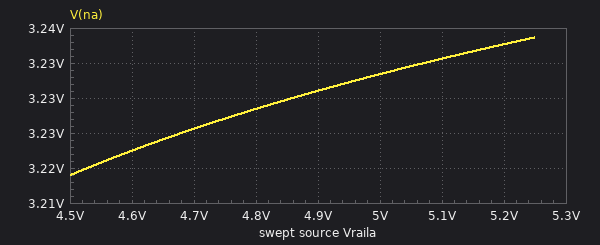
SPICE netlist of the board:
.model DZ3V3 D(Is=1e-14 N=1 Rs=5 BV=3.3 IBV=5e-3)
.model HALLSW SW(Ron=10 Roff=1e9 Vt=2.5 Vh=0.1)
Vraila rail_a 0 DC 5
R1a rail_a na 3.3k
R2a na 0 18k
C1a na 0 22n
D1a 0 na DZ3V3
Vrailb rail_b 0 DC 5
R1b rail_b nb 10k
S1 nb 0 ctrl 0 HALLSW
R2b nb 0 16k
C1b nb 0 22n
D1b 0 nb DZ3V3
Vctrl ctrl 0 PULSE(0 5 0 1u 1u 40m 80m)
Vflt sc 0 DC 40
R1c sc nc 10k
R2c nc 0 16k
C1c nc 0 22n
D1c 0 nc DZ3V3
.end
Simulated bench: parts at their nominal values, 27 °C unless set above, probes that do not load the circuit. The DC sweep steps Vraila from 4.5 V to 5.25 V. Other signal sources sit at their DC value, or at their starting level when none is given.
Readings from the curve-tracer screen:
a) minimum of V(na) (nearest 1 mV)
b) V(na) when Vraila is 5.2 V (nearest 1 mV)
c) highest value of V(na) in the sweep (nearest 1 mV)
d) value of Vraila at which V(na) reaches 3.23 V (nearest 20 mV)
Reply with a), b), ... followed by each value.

a) 3.219 V
b) 3.238 V
c) 3.239 V
d) 4.68 V
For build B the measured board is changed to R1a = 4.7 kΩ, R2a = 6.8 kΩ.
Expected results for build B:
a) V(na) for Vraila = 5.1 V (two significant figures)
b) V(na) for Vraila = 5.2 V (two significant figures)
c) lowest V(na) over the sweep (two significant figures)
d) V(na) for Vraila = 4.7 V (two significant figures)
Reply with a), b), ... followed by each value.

a) 3.0 V
b) 3.1 V
c) 2.7 V
d) 2.8 V
